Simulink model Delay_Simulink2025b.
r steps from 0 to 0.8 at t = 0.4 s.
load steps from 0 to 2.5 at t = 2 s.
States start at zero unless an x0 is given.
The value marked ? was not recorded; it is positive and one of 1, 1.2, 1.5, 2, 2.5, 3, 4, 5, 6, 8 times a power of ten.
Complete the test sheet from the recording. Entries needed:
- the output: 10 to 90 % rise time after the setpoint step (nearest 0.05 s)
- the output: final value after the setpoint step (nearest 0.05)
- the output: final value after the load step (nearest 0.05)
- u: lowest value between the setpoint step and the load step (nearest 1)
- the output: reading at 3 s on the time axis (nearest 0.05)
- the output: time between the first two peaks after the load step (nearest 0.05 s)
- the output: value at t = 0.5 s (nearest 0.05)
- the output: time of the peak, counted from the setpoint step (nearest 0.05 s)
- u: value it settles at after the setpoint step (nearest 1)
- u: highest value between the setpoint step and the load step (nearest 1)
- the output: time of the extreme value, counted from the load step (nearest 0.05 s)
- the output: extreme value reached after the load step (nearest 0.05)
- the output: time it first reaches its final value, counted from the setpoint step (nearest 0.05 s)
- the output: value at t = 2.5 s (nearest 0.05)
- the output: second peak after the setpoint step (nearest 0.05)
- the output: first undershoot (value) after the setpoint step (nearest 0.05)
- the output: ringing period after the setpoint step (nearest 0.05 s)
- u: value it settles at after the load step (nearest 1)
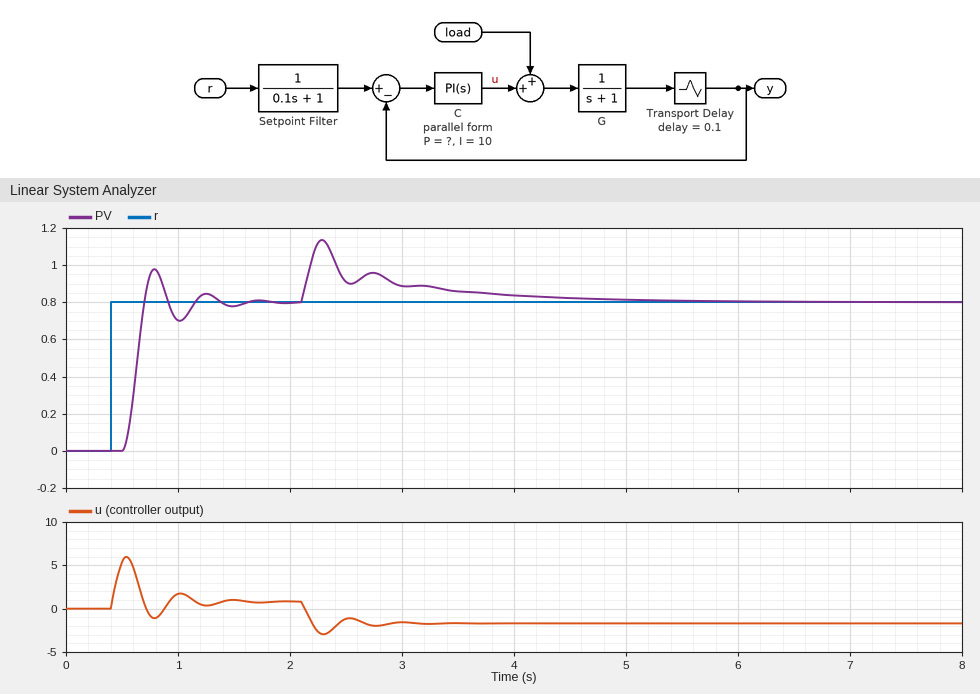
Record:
0.15 s
0.80
0.80
-1
0.90
0.45 s
0.00
0.40 s
1
6
0.30 s
1.15
0.30 s
0.90
0.85
0.70
0.45 s
-2
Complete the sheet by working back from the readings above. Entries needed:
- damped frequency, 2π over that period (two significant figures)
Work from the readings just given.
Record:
14 rad/s
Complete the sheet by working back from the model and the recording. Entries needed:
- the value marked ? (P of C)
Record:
10
